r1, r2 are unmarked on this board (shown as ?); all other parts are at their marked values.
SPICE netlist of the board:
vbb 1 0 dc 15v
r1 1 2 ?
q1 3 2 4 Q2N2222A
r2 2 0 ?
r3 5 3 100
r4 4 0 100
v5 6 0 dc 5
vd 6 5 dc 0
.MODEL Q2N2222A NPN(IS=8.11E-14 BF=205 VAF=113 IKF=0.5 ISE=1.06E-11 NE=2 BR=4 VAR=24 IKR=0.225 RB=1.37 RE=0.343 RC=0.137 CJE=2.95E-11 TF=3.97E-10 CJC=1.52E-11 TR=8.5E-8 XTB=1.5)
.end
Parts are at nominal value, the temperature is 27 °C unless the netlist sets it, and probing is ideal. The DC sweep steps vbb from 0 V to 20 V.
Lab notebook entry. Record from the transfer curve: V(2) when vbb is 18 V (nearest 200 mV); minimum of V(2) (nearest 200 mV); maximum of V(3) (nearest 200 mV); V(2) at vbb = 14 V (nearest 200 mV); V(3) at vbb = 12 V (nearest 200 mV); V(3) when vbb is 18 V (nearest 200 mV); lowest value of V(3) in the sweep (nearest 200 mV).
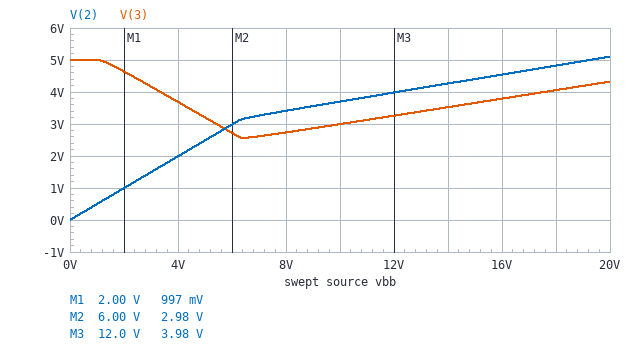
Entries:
4.8 V
0 V
5.0 V
4.2 V
3.2 V
4.0 V
2.6 V
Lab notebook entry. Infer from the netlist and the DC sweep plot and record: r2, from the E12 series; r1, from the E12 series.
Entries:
270 Ω
270 Ω
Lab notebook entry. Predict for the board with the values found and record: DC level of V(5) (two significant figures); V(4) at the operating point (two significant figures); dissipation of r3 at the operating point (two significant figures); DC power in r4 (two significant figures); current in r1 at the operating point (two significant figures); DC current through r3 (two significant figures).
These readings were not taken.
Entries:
5.0 V
3.6 V
18 mW
130 mW
39 mA
13 mA
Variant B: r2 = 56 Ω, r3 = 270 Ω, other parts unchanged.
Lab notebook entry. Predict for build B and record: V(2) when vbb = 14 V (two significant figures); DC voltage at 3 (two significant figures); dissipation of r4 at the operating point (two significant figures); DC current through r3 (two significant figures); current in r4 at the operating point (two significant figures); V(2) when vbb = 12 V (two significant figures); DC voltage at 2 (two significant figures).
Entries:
2.3 V
1.7 V
28 mW
12 mA
17 mA
2.0 V
2.4 V
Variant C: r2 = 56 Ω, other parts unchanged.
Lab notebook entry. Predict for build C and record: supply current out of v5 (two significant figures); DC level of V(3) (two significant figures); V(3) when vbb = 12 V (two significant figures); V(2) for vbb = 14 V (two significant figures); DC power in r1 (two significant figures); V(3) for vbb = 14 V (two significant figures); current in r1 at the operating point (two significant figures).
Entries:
19 mA
3.1 V
3.6 V
2.4 V
570 mW
3.3 V
46 mA
